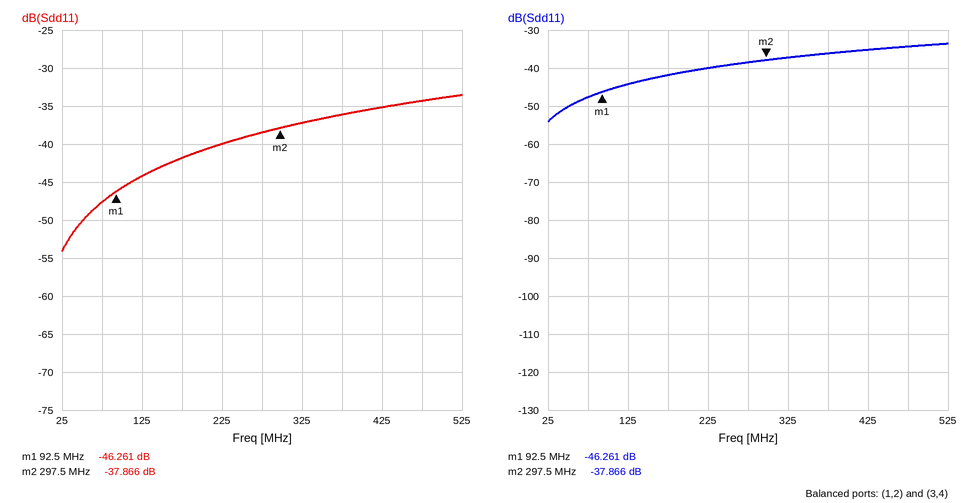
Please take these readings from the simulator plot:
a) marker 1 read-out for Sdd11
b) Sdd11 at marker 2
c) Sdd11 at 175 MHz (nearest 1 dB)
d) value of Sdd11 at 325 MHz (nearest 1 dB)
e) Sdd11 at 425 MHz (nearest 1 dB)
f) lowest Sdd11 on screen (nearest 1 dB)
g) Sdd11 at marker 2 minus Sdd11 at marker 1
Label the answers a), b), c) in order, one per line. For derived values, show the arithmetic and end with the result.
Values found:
a) -46.261 dB
b) -37.866 dB
c) -42 dB
d) -37 dB
e) -35 dB
f) -54 dB
g) -37.866 − (-46.261) = 8.395 dB
